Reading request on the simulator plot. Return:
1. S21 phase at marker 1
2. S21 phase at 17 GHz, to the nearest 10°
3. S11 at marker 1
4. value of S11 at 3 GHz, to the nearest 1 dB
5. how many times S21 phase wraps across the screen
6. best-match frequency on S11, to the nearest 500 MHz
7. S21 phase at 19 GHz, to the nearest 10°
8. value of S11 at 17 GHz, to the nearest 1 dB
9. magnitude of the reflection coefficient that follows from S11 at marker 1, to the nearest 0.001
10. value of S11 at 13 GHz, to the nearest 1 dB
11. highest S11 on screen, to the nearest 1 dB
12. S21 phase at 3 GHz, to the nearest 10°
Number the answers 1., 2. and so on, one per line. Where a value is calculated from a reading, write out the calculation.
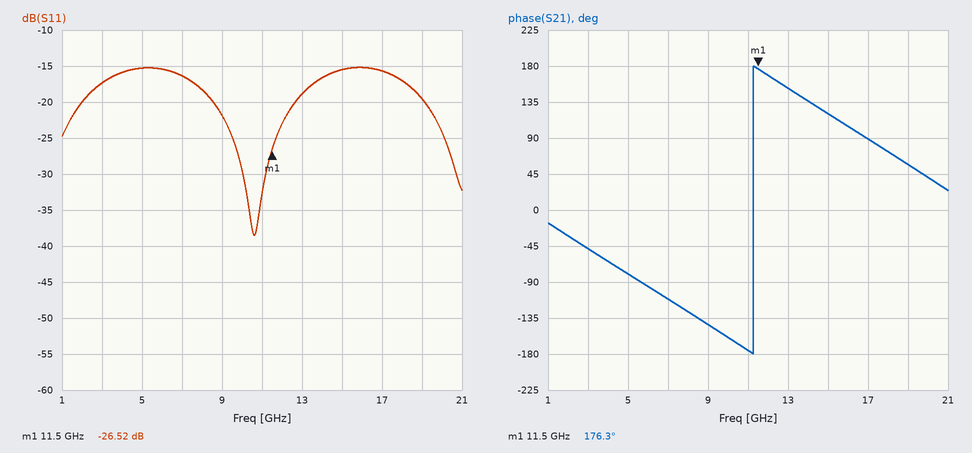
1. 176.3°
2. 90°
3. -26.52 dB
4. -17 dB
5. 1
6. 10.5 GHz
7. 60°
8. -16 dB
9. 10^(-26.52/20) ≈ 0.047
10. -19 dB
11. -15 dB
12. -50°
